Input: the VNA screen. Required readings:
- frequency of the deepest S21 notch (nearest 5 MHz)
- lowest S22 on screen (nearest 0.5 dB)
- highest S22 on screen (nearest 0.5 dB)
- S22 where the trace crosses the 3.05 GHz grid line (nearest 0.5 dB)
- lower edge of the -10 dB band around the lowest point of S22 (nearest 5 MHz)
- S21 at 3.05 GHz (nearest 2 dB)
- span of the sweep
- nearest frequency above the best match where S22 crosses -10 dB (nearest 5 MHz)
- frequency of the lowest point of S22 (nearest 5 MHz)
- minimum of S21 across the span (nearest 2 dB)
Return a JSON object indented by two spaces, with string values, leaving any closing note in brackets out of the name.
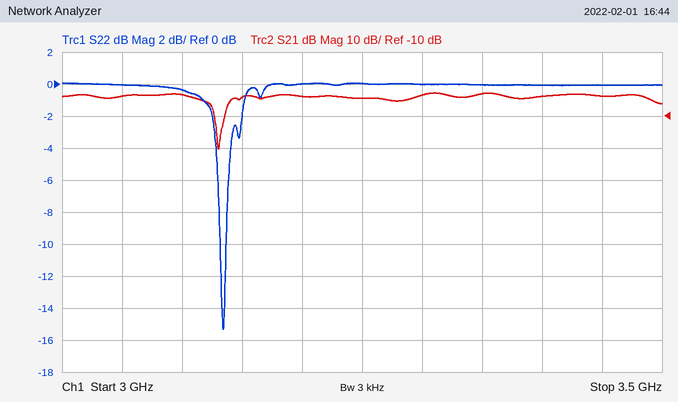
{
  "frequency of the deepest S21 notch": "3.130 GHz",
  "lowest S22 on screen": "-15.5 dB",
  "highest S22 on screen": "0.0 dB",
  "S22 where the trace crosses the 3.05 GHz grid line": "0.0 dB",
  "lower edge of the -10 dB band around the lowest point of S22": "3.130 GHz",
  "S21 at 3.05 GHz": "-4 dB",
  "span of the sweep": "500 MHz",
  "nearest frequency above the best match where S22 crosses -10 dB": "3.135 GHz",
  "frequency of the lowest point of S22": "3.135 GHz",
  "minimum of S21 across the span": "-20 dB"
}
